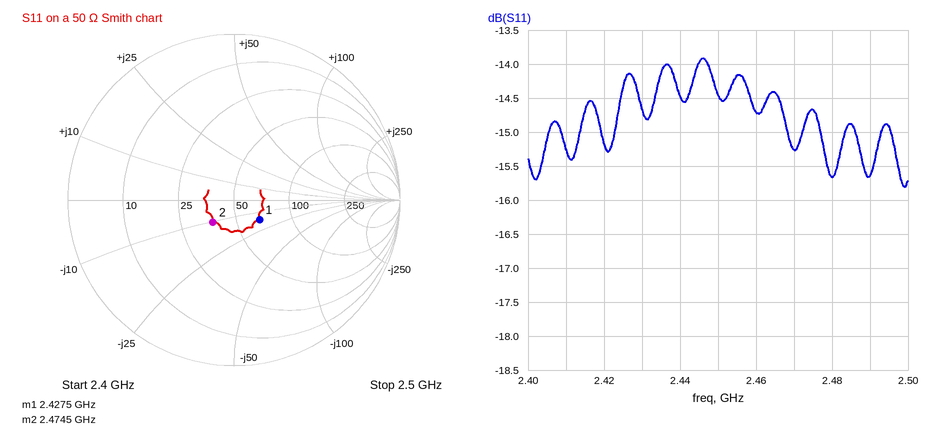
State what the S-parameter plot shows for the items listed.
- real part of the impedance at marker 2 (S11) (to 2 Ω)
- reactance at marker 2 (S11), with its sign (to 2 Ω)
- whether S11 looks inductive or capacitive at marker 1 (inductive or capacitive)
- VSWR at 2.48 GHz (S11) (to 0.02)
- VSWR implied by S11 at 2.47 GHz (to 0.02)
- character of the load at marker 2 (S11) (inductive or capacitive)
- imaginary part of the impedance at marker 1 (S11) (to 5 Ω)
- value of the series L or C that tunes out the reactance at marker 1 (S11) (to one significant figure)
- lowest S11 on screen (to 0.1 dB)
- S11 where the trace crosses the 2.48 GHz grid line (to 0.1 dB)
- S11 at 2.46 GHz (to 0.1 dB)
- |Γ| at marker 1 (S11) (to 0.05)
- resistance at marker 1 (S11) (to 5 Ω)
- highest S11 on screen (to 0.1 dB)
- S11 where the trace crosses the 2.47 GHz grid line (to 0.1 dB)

38 Ω
-10 Ω
capacitive
1.40
1.42
capacitive
-15 Ω
1 nH
-15.8 dB
-15.7 dB
-14.7 dB
0.20
65 Ω
-13.9 dB
-15.3 dB
